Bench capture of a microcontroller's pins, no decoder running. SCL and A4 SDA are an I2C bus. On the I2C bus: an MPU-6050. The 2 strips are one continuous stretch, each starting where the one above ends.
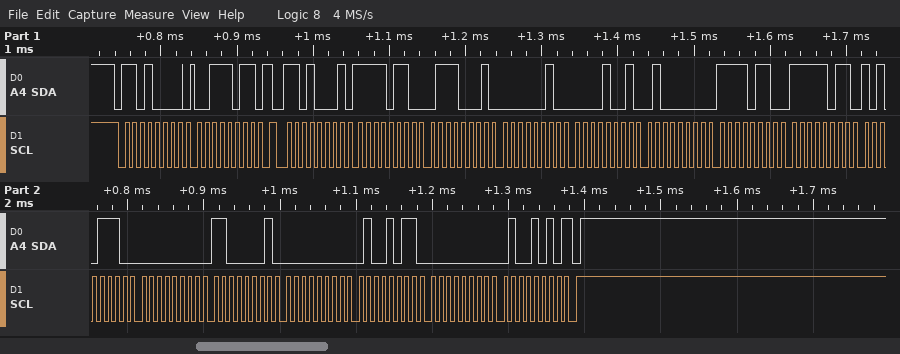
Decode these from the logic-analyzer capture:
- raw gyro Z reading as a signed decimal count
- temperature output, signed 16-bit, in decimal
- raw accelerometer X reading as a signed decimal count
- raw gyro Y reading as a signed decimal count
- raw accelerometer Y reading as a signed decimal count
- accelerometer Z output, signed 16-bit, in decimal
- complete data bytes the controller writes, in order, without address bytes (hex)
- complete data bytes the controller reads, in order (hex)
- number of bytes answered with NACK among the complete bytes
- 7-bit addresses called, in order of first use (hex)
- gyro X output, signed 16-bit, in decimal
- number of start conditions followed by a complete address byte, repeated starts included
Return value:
74
-1106
-2447
75
521
16630
3B
F6 71 02 09 40 F6 FB AE 00 C1 00 4B 00 4A
1
0x68
193
2
